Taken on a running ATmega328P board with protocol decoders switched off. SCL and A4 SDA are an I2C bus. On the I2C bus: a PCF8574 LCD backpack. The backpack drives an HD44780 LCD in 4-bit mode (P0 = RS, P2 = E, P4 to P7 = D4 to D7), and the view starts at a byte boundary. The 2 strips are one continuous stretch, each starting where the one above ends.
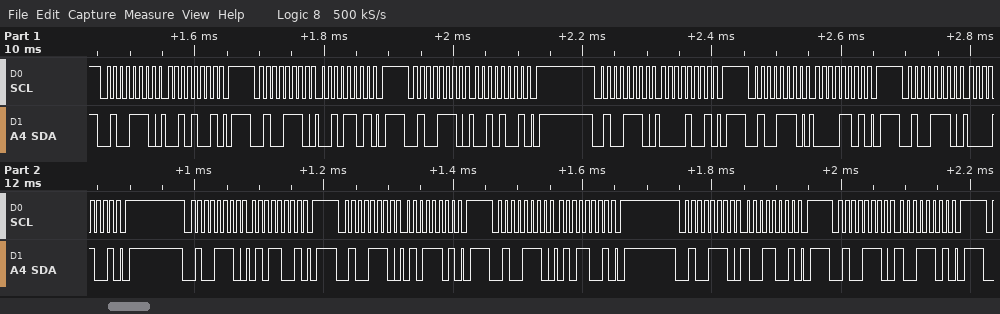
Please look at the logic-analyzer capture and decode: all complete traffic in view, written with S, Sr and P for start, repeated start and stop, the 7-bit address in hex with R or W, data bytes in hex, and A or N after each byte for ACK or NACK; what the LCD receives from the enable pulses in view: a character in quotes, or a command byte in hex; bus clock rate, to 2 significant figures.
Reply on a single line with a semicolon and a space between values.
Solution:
S 27W A 29 A P S 27W A 2D A P S 27W A 29 A P S 27W A 09 A P S 27W A 0D A P S 27W A 09 A P S 27W A 59 A P S 27W A 5D A P S 27W A 59 A P S 27W A 99 A P S 27W A 9D A P; ' '; 100 kHz
